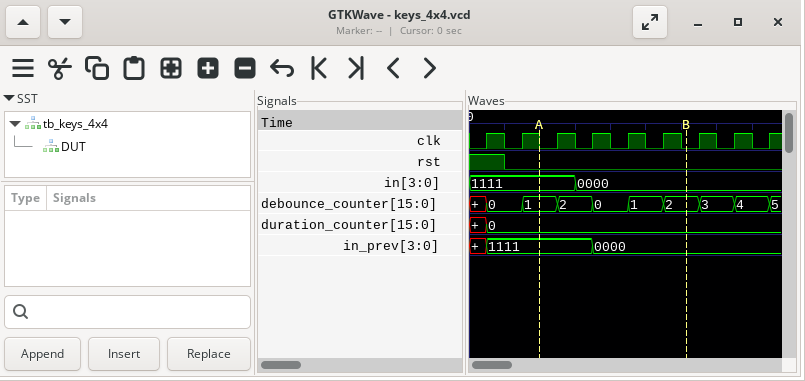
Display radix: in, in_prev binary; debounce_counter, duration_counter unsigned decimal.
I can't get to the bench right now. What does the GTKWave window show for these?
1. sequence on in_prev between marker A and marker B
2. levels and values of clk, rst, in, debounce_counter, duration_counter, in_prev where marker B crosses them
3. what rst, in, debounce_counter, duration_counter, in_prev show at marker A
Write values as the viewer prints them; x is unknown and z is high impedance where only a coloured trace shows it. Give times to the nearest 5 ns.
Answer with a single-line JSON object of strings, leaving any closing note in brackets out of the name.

{"sequence on in_prev between marker A and marker B": "1111, 0000", "levels and values of clk, rst, in, debounce_counter, duration_counter, in_prev where marker B crosses them": "clk=0, rst=0, in=0000, debounce_counter=2, duration_counter=0, in_prev=0000", "what rst, in, debounce_counter, duration_counter, in_prev show at marker A": "rst=0, in=1111, debounce_counter=1, duration_counter=0, in_prev=1111"}
